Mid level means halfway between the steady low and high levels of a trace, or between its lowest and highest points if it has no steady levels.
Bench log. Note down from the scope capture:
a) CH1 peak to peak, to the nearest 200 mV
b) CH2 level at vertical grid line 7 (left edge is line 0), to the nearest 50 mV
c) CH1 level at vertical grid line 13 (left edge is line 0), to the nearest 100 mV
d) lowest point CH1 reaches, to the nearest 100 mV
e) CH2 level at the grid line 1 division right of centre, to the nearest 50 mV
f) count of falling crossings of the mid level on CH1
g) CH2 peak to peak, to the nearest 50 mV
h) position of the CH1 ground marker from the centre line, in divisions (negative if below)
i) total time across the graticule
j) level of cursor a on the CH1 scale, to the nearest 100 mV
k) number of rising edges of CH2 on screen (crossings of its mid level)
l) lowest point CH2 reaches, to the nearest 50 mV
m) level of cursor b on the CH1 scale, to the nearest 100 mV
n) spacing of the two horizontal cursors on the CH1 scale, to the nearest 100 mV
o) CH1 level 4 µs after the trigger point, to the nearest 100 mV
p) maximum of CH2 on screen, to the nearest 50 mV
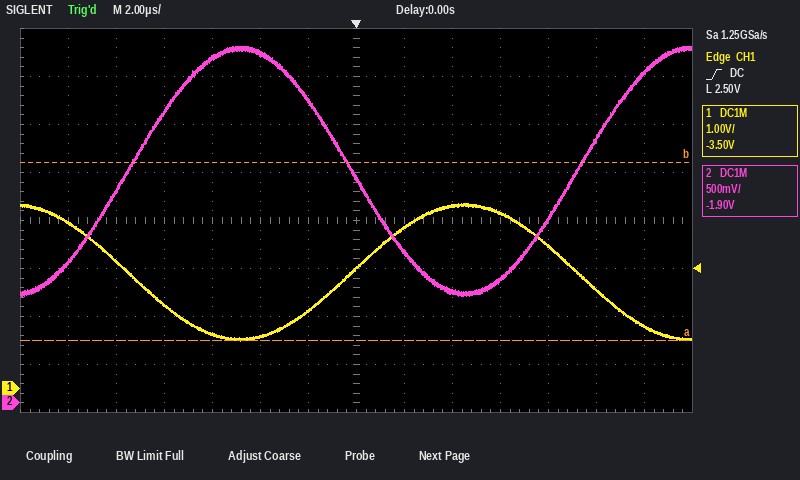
2.8 V
2.35 V
1.3 V
1.0 V
1.55 V
2
2.60 V
-3.5 div
28 µs
1.0 V
2
1.10 V
4.7 V
3.7 V
3.8 V
3.70 V
